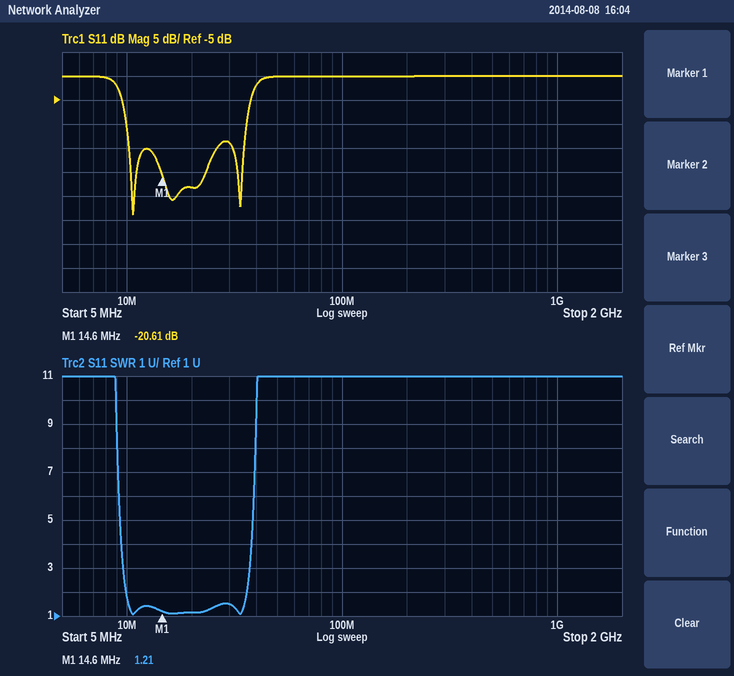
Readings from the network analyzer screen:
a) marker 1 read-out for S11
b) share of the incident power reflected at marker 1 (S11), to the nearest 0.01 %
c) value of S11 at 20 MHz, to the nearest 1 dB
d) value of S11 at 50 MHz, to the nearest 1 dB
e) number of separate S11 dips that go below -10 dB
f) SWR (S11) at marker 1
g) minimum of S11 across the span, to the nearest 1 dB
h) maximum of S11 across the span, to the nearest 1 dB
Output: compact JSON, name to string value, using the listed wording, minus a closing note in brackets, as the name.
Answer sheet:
{"marker 1 read-out for S11": "-20.61 dB", "share of the incident power reflected at marker 1 (S11), to the nearest 0.01 %": "0.87 %", "value of S11 at 20 MHz, to the nearest 1 dB": "-23 dB", "value of S11 at 50 MHz, to the nearest 1 dB": "0 dB", "number of separate S11 dips that go below -10 dB": "3", "SWR (S11) at marker 1": "1.21", "minimum of S11 across the span, to the nearest 1 dB": "-29 dB", "maximum of S11 across the span, to the nearest 1 dB": "0 dB"}
